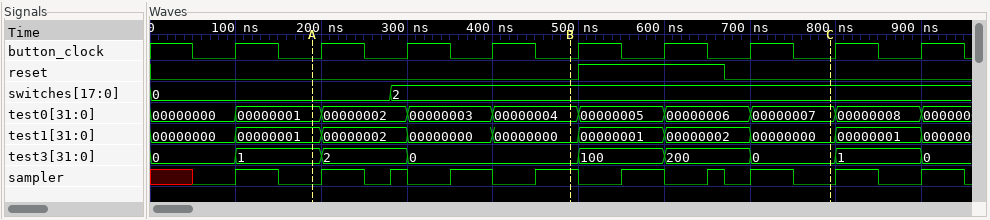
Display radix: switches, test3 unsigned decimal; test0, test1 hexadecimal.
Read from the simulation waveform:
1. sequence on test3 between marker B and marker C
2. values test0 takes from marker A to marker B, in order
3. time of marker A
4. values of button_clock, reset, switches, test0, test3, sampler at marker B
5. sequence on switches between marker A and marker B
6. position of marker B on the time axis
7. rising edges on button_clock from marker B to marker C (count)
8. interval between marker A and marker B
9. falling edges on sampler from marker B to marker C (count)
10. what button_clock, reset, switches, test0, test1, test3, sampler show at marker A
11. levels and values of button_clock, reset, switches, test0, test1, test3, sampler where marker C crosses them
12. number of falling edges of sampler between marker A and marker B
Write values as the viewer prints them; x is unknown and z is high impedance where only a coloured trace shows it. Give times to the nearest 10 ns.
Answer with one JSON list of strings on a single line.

["0, 100, 200, 0", "00000001, 00000002, 00000003, 00000004", "190 ns", "button_clock=0, reset=0, switches=2, test0=00000004, test3=0, sampler=1", "0, 2", "490 ns", "3", "300 ns", "4", "button_clock=0, reset=0, switches=0, test0=00000001, test1=00000001, test3=1, sampler=0", "button_clock=0, reset=0, switches=2, test0=00000007, test1=00000000, test3=0, sampler=0", "3"]
